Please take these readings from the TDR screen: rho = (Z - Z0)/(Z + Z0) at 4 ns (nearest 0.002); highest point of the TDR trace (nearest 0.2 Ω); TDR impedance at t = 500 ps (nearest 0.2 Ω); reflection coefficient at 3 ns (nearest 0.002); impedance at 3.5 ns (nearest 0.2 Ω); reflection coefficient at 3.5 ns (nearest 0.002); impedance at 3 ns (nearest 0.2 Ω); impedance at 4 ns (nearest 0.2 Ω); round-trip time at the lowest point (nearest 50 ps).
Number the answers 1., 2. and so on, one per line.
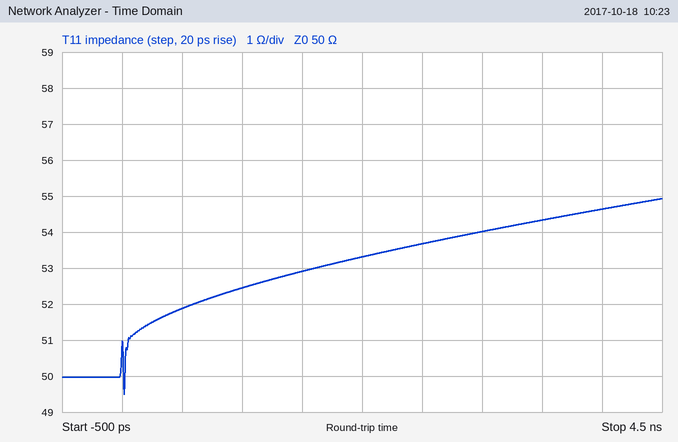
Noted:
1. +0.044
2. 55.0 Ω
3. 51.8 Ω
4. +0.038
5. 54.4 Ω
6. +0.042
7. 54.0 Ω
8. 54.6 Ω
9. 0 ps
